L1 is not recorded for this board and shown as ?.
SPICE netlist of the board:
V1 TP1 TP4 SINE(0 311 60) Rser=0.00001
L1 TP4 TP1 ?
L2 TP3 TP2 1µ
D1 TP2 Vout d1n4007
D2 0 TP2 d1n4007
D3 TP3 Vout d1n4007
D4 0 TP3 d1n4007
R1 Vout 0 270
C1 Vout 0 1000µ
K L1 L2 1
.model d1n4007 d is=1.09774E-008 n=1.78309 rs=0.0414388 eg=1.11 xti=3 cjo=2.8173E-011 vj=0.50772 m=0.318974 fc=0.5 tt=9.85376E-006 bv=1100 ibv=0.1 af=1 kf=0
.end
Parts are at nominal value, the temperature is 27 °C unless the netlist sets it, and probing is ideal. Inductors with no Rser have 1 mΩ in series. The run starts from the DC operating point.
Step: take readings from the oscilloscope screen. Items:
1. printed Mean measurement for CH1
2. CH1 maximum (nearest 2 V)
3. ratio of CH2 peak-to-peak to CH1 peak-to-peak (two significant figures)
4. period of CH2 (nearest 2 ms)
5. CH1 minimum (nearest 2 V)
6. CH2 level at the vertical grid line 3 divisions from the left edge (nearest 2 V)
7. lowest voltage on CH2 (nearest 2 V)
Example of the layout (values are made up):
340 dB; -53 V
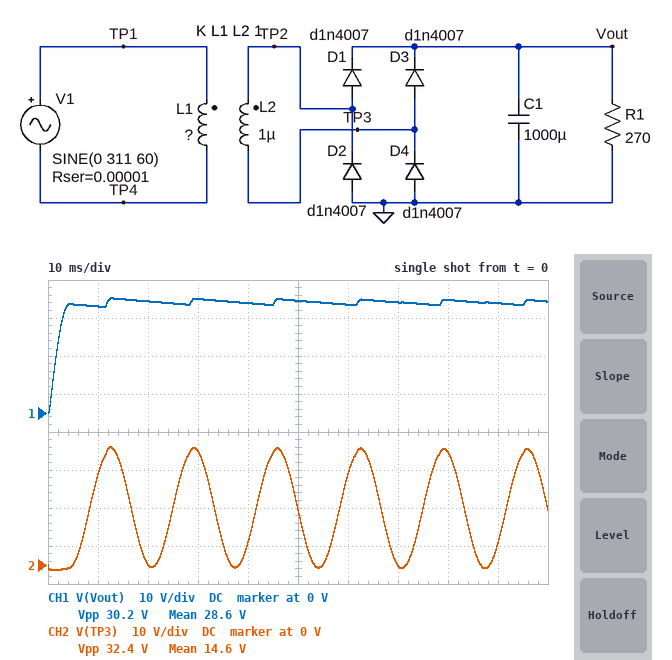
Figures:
28.6 V; 30 V; 1.1; 16 ms; 0 V; 30 V; -2 V
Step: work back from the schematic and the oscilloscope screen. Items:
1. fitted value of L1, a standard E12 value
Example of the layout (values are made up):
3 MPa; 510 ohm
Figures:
100 µH
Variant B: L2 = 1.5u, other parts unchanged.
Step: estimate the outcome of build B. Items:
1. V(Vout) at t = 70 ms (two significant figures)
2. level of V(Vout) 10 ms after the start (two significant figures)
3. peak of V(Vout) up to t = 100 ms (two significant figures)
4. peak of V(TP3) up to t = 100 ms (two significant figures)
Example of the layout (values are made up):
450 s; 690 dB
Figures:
36 V; 35 V; 37 V; 38 V
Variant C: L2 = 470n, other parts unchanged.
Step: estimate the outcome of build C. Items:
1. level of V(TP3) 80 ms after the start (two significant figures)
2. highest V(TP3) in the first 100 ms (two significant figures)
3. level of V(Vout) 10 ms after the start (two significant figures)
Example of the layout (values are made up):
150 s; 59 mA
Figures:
20 V; 21 V; 19 V
